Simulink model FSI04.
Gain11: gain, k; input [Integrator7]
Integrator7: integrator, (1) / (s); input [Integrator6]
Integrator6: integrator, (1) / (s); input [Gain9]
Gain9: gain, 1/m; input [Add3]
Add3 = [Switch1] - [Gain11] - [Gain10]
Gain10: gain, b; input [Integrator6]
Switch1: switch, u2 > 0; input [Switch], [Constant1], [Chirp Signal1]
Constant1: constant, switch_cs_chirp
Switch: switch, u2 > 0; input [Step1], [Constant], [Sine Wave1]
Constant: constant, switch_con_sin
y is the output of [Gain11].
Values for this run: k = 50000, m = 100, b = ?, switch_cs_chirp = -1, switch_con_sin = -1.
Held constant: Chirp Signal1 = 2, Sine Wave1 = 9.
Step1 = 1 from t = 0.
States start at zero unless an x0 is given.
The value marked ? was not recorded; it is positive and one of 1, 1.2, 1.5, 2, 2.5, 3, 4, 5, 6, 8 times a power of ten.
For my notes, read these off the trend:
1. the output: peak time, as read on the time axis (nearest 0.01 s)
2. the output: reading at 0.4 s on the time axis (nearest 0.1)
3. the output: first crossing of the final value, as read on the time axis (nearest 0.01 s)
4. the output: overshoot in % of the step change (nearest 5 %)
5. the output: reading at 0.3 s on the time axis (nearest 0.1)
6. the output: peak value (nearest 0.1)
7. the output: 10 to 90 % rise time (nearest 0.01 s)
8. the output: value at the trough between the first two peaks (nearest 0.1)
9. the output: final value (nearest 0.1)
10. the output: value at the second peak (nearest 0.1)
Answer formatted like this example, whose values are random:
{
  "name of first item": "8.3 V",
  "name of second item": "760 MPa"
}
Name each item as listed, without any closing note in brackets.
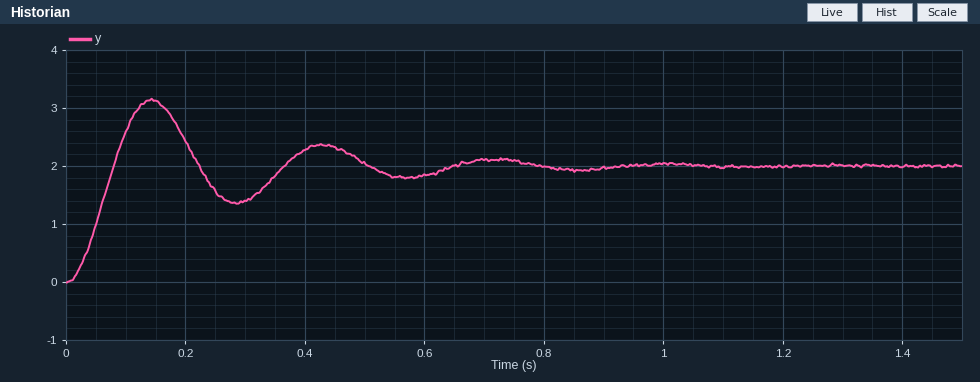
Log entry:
{
  "the output: peak time, as read on the time axis": "0.14 s",
  "the output: reading at 0.4 s on the time axis": "2.3",
  "the output: first crossing of the final value, as read on the time axis": "0.08 s",
  "the output: overshoot in % of the step change": "55 %",
  "the output: reading at 0.3 s on the time axis": "1.4",
  "the output: peak value": "3.1",
  "the output: 10 to 90 % rise time": "0.05 s",
  "the output: value at the trough between the first two peaks": "1.4",
  "the output: final value": "2.0",
  "the output: value at the second peak": "2.4"
}
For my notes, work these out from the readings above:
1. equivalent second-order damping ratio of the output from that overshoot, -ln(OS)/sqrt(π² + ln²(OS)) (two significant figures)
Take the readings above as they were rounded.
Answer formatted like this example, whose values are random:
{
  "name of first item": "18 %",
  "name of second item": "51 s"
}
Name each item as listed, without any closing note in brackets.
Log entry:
{
  "equivalent second-order damping ratio of the output from that overshoot, -ln(OS)/sqrt(π² + ln²(OS))": "0.19"
}
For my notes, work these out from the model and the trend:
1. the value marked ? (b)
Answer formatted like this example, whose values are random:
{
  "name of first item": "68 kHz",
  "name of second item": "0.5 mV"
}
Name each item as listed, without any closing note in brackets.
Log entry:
{
  "the value marked ?": "800"
}
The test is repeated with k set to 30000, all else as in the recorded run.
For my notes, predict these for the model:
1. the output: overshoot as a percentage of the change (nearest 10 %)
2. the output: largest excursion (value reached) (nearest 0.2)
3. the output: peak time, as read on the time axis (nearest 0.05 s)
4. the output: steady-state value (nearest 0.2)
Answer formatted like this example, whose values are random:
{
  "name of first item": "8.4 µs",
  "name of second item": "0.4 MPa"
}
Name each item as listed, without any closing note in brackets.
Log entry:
{
  "the output: overshoot as a percentage of the change": "50 %",
  "the output: largest excursion (value reached)": "3.0",
  "the output: peak time, as read on the time axis": "0.20 s",
  "the output: steady-state value": "2.0"
}
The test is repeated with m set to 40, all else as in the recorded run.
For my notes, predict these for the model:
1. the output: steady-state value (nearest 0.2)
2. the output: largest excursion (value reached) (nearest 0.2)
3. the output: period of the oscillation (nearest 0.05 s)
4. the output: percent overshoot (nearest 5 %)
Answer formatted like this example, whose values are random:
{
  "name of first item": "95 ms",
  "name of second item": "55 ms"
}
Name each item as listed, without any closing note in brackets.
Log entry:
{
  "the output: steady-state value": "2.0",
  "the output: largest excursion (value reached)": "2.8",
  "the output: period of the oscillation": "0.20 s",
  "the output: percent overshoot": "40 %"
}
